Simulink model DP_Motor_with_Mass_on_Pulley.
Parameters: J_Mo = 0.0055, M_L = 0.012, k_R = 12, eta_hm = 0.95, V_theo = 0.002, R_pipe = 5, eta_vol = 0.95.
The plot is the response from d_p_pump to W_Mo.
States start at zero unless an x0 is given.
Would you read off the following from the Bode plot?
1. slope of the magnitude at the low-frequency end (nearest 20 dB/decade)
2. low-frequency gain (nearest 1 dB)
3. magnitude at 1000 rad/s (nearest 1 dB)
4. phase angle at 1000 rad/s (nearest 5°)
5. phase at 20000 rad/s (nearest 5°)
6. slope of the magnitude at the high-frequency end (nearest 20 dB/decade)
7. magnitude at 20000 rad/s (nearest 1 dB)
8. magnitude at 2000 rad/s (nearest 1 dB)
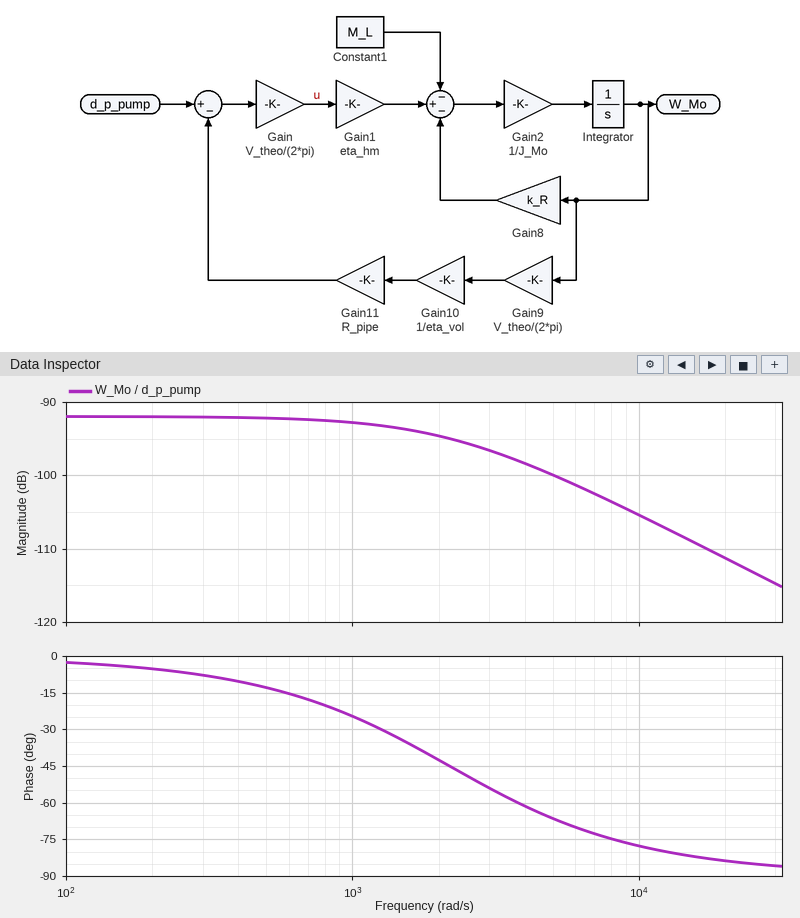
0 dB/decade
-92 dB
-93 dB
-25°
-85°
-20 dB/decade
-111 dB
-95 dB
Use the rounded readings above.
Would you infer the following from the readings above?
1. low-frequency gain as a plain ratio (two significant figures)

0.000025
